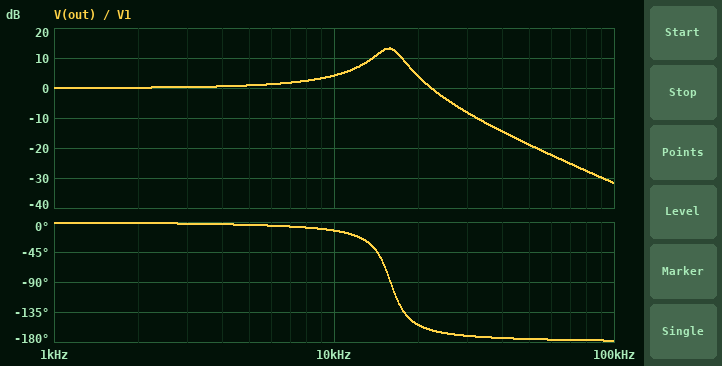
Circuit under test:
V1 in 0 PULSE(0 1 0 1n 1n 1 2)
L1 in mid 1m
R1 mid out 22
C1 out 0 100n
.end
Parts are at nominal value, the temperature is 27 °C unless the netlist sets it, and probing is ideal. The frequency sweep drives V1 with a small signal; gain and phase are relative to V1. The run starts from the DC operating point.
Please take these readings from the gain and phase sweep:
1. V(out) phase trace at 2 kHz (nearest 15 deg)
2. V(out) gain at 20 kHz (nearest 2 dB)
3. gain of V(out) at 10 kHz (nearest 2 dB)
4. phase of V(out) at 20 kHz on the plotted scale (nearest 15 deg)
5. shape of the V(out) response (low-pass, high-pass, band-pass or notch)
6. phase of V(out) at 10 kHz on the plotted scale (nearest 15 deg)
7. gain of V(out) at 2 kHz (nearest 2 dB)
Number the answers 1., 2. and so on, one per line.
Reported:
1. 0 deg
2. 4 dB
3. 4 dB
4. -150 deg
5. low-pass
6. -15 deg
7. 0 dB
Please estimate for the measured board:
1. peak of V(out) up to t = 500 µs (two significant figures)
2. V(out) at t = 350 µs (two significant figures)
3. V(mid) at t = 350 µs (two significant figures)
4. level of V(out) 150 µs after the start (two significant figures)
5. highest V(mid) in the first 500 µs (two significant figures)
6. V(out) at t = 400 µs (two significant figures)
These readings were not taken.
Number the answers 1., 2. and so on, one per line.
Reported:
1. 1.7 V
2. 1.0 V
3. 1.0 V
4. 1.1 V
5. 1.7 V
6. 1.0 V
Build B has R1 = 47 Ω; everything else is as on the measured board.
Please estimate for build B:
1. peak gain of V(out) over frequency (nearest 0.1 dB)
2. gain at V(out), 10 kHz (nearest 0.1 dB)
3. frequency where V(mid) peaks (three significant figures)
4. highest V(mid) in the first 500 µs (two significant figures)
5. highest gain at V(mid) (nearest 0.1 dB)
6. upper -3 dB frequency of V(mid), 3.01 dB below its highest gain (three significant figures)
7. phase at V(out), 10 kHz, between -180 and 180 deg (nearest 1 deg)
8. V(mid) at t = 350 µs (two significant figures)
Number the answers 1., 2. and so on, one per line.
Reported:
1. 6.8 dB
2. 3.4 dB
3. 15.2 kHz
4. 1.5 V
5. 7.6 dB
6. 18.7 kHz
7. -26 deg
8. 1.0 V
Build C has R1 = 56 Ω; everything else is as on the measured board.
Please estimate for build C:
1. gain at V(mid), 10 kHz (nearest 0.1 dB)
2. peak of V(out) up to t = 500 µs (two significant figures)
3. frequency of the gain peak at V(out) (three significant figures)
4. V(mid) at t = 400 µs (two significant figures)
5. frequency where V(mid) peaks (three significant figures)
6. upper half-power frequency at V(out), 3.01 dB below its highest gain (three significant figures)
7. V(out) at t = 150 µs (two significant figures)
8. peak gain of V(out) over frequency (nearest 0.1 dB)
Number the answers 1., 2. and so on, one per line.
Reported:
1. 3.6 dB
2. 1.4 V
3. 14.6 kHz
4. 1.0 V
5. 14.9 kHz
6. 18.7 kHz
7. 1.0 V
8. 5.4 dB
